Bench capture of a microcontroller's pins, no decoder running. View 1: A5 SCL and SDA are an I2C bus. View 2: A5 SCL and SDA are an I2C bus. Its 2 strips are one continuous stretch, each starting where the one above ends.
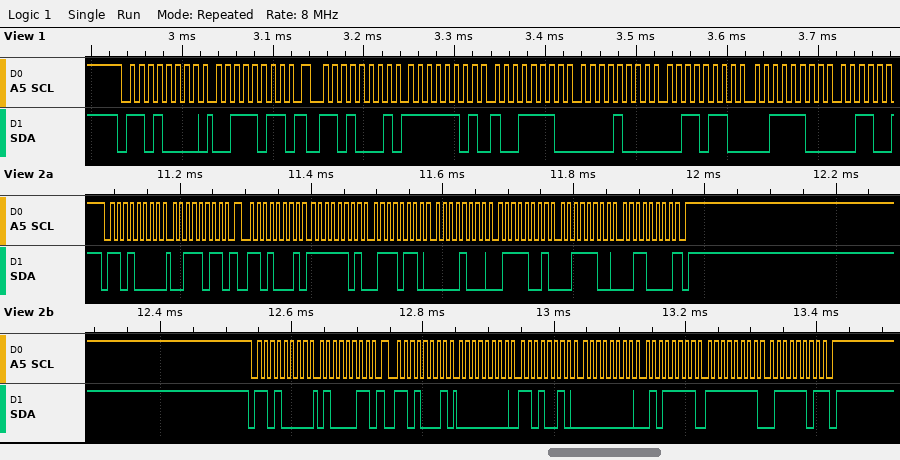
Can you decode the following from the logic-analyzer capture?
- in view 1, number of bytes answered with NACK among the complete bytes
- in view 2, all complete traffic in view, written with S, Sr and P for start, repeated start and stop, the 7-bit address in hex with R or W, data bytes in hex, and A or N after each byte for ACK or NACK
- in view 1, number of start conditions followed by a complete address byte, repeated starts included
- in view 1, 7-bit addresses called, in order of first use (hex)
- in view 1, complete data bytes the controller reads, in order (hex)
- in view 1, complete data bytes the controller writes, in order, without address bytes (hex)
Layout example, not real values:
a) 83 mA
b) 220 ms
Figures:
a) 0
b) S 68W A 3B A Sr 68R A FD A 76 A 08 A 79 A 3C A 30 N P S 68W A 43 A Sr 68R A 00 A D2 A 00 A 5F A FF A 7D N P
c) 2
d) 0x68
e) FD 9E 08 36 3C
f) 3B
